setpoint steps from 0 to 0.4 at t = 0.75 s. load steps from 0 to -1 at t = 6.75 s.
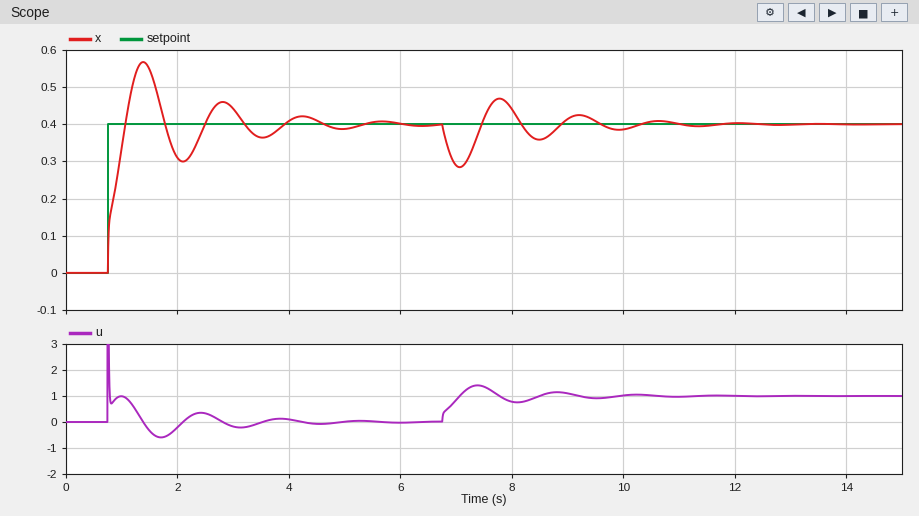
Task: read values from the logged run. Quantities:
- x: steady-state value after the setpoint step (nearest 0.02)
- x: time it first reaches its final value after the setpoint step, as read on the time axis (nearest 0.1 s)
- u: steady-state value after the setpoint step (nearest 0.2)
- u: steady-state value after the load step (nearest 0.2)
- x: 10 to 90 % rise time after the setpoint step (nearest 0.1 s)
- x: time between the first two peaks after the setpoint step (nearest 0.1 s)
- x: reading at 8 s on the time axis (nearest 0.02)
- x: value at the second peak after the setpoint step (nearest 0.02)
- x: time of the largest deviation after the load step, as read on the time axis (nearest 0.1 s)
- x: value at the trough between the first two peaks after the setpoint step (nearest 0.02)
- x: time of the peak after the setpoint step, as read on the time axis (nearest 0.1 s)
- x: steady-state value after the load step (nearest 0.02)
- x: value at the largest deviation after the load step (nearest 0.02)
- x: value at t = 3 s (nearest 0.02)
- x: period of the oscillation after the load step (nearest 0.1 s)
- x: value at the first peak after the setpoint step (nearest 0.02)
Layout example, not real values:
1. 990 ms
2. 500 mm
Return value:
1. 0.40
2. 1.1 s
3. 0.0
4. 1.0
5. 0.3 s
6. 1.4 s
7. 0.44
8. 0.46
9. 7.1 s
10. 0.30
11. 1.4 s
12. 0.40
13. 0.28
14. 0.44
15. 1.4 s
16. 0.56
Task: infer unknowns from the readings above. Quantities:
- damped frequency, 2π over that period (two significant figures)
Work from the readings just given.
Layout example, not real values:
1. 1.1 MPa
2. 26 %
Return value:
1. 4.5 rad/s
